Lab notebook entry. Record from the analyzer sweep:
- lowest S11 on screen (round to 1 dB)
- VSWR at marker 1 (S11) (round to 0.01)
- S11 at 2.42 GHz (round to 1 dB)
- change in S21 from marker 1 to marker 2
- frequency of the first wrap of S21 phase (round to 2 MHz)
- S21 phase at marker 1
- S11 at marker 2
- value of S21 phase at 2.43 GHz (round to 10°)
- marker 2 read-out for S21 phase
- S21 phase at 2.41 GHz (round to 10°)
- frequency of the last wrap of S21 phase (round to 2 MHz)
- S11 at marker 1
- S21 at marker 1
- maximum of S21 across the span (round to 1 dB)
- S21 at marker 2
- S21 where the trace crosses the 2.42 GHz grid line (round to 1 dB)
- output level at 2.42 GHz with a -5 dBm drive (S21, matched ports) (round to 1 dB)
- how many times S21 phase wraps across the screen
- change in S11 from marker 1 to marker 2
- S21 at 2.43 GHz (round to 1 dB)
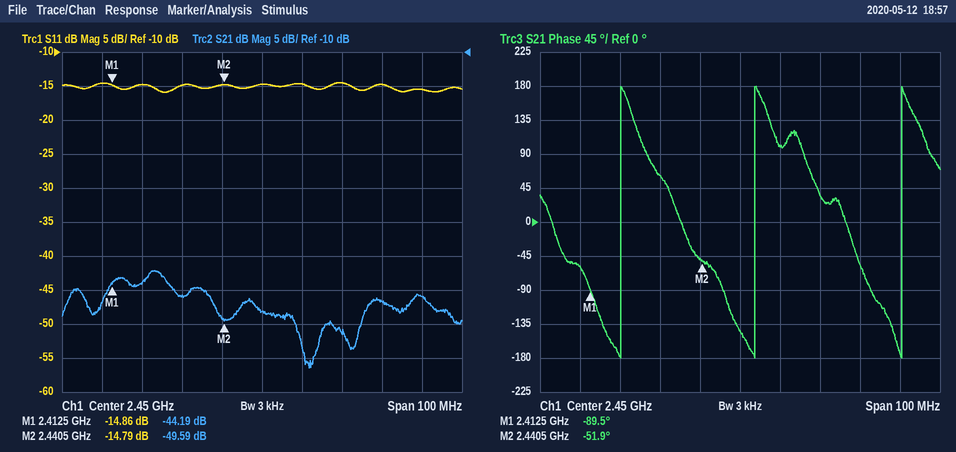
-16 dB
1.44
-15 dB
-5.40 dB
2.420 GHz
-89.5°
-14.79 dB
60°
-51.9°
-60°
2.490 GHz
-14.86 dB
-44.19 dB
-42 dB
-49.59 dB
-44 dB
-49 dBm
3
0.07 dB
-46 dB
